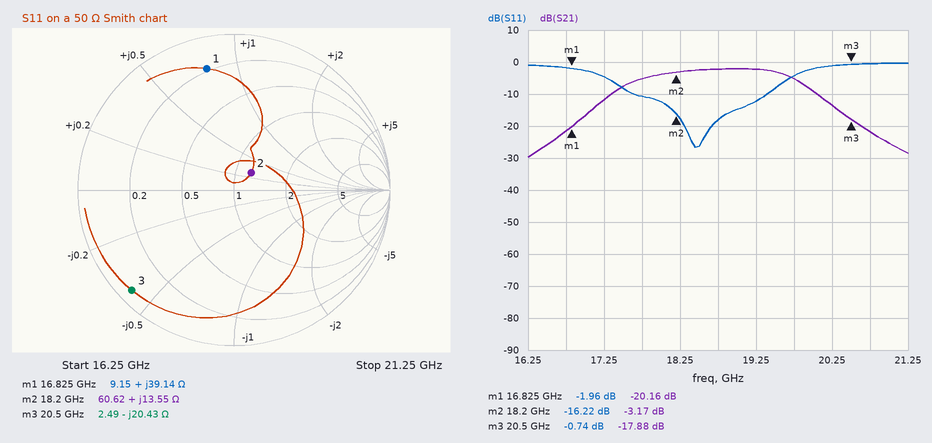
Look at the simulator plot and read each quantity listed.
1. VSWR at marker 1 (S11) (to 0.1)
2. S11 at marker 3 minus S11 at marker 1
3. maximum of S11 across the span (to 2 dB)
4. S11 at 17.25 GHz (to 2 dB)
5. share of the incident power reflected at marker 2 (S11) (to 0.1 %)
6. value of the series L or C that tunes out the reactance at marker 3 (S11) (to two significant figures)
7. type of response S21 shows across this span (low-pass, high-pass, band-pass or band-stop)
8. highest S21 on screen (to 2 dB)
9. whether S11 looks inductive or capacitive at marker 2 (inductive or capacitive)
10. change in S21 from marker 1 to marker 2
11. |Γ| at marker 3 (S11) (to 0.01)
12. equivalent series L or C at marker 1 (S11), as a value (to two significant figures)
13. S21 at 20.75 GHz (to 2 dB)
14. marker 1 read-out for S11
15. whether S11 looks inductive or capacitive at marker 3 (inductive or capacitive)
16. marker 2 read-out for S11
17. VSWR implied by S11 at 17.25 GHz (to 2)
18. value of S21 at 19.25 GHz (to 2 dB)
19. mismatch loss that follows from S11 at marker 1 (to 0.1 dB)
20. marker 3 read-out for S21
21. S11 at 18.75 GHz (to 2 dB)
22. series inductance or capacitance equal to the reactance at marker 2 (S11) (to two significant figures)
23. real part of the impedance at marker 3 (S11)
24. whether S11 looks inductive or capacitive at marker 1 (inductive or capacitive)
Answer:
8.9
1.22 dB
0 dB
-4 dB
2.4 %
160 pH
band-pass
-2 dB
inductive
16.99 dB
0.92
370 pH
-22 dB
-1.96 dB
capacitive
-16.22 dB
4
-2 dB
4.4 dB
-17.88 dB
-18 dB
120 pH
2.49 Ω
inductive
